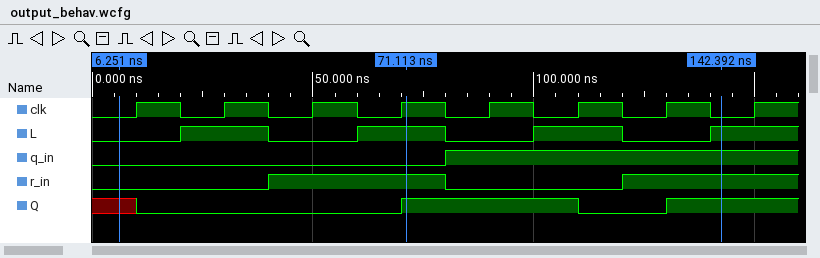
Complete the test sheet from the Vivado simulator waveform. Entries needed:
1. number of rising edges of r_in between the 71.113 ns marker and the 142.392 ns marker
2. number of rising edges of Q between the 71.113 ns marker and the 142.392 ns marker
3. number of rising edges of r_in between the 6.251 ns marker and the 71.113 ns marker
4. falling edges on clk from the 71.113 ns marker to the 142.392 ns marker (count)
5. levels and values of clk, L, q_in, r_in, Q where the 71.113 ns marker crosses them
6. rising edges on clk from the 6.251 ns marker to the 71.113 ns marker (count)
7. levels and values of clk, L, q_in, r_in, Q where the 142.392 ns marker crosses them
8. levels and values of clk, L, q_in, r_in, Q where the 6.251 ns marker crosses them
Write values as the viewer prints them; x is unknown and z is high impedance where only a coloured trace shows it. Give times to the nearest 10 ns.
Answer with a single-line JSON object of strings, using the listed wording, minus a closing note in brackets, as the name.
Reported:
{"number of rising edges of r_in between the 71.113 ns marker and the 142.392 ns marker": "1", "number of rising edges of Q between the 71.113 ns marker and the 142.392 ns marker": "1", "number of rising edges of r_in between the 6.251 ns marker and the 71.113 ns marker": "1", "falling edges on clk from the 71.113 ns marker to the 142.392 ns marker": "4", "levels and values of clk, L, q_in, r_in, Q where the 71.113 ns marker crosses them": "clk=1, L=1, q_in=0, r_in=1, Q=1", "rising edges on clk from the 6.251 ns marker to the 71.113 ns marker": "4", "levels and values of clk, L, q_in, r_in, Q where the 142.392 ns marker crosses them": "clk=0, L=1, q_in=1, r_in=1, Q=1", "levels and values of clk, L, q_in, r_in, Q where the 6.251 ns marker crosses them": "clk=0, L=0, q_in=0, r_in=0, Q=x"}
